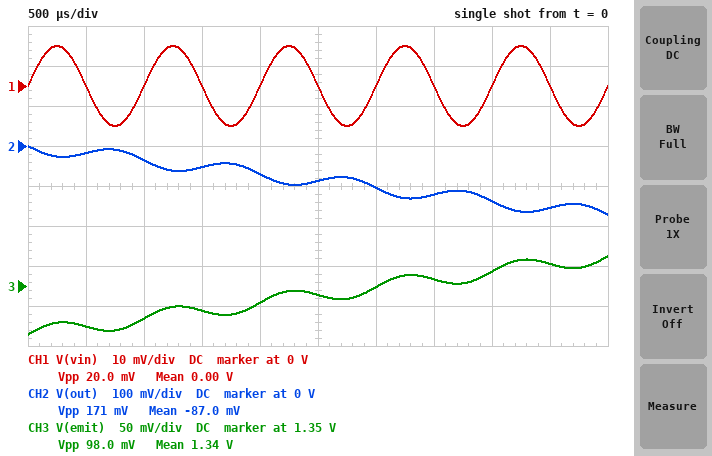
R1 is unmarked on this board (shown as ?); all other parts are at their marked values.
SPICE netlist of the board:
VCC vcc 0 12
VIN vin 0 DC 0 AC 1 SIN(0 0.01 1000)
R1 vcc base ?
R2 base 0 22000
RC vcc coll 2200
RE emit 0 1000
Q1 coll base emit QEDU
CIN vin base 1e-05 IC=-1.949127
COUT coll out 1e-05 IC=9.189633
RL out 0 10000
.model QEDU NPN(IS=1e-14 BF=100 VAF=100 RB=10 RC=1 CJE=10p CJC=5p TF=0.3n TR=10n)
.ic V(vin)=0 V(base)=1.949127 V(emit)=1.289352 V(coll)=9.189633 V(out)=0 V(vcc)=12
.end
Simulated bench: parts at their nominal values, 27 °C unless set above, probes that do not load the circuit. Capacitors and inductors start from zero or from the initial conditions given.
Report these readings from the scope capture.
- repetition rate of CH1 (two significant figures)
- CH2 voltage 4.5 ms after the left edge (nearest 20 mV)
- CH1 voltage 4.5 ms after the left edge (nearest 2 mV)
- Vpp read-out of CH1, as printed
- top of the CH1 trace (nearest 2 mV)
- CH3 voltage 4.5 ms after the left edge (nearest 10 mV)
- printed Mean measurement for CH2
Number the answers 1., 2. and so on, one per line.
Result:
1. 1.0 kHz
2. -160 mV
3. 0 V
4. 20.0 mV
5. 10 mV
6. 1.38 V
7. -87.0 mV
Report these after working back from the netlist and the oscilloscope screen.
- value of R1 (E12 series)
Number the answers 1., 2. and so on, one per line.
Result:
1. 33 kΩ
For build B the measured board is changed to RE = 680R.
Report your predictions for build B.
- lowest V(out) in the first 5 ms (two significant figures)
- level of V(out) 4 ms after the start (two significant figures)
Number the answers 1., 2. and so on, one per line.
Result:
1. -1.3 V
2. -1.2 V
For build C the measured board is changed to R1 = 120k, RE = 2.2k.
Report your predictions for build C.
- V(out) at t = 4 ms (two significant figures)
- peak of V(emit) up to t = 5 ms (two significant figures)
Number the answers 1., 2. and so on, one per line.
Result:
1. 1.2 V
2. 1.3 V
